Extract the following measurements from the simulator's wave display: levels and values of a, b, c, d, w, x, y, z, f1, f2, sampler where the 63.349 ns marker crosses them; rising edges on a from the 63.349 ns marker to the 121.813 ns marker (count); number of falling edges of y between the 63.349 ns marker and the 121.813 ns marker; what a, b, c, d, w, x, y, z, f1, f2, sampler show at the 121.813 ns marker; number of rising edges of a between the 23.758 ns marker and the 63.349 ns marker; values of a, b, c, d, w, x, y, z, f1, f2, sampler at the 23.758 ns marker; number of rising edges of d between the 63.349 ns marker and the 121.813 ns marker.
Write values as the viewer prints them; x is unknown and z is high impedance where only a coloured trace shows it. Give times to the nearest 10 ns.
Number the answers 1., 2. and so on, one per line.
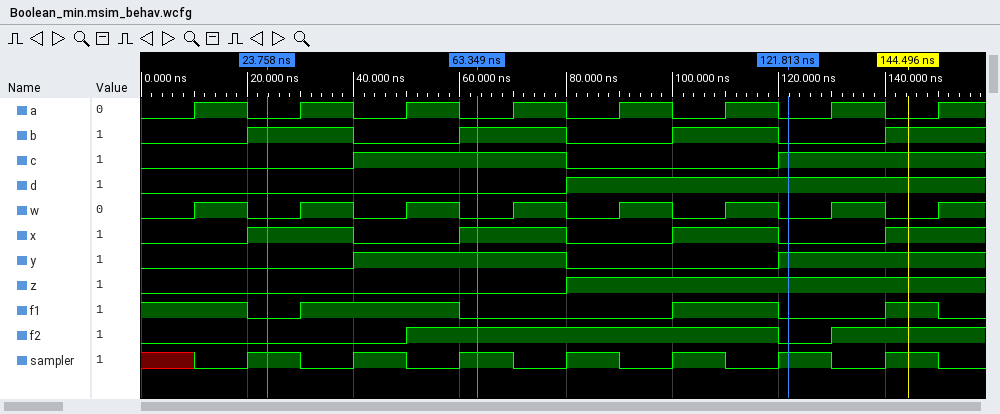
1. a=0, b=1, c=1, d=0, w=0, x=1, y=1, z=0, f1=0, f2=1, sampler=1
2. 3
3. 1
4. a=0, b=0, c=1, d=1, w=0, x=0, y=1, z=1, f1=0, f2=0, sampler=1
5. 2
6. a=0, b=1, c=0, d=0, w=0, x=1, y=0, z=0, f1=0, f2=0, sampler=1
7. 1
